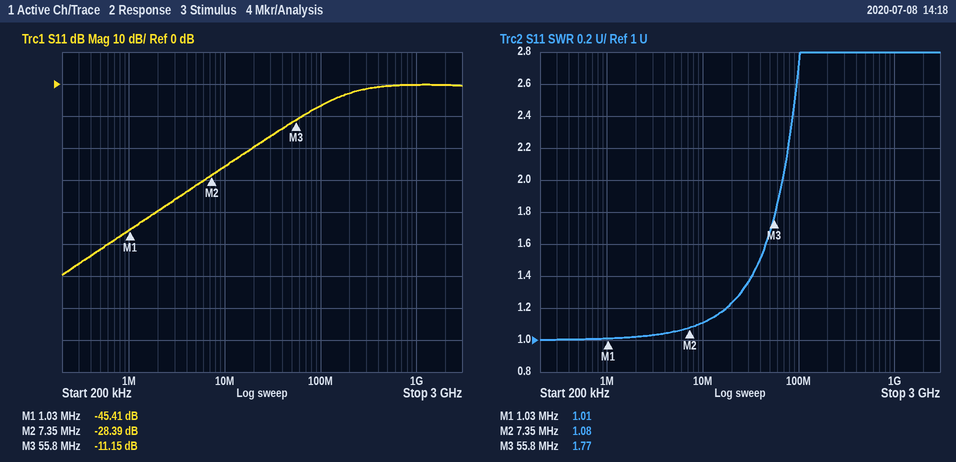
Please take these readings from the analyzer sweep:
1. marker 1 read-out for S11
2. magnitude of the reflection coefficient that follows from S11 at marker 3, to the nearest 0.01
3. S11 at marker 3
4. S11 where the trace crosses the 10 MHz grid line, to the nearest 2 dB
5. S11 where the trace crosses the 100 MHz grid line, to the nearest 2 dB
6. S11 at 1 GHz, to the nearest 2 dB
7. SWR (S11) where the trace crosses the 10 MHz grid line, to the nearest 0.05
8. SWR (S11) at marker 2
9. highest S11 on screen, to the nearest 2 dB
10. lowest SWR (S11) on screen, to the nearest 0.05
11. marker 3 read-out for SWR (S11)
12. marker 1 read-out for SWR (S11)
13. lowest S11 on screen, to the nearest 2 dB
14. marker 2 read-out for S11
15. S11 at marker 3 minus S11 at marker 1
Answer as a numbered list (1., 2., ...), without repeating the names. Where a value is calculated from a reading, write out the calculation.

1. -45.41 dB
2. 10^(-11.15/20) ≈ 0.28
3. -11.15 dB
4. -26 dB
5. -6 dB
6. 0 dB
7. 1.10
8. 1.08
9. 0 dB
10. 1.00
11. 1.77
12. 1.01
13. -60 dB
14. -28.39 dB
15. -11.15 − (-45.41) = 34.26 dB
